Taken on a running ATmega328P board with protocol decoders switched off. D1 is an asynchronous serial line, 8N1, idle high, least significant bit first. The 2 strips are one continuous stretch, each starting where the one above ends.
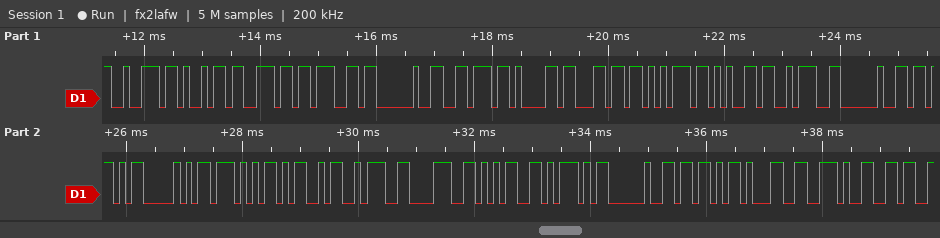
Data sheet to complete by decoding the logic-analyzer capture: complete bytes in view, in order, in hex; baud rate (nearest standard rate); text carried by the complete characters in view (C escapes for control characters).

72 69 6E 67 20 76 61 6C 75 65 3A 20 5B 50 57 4D 3A 38 35 5D 20 5B 31 2E 36
9600 baud
"ring value: [PWM:85] [1.6"
